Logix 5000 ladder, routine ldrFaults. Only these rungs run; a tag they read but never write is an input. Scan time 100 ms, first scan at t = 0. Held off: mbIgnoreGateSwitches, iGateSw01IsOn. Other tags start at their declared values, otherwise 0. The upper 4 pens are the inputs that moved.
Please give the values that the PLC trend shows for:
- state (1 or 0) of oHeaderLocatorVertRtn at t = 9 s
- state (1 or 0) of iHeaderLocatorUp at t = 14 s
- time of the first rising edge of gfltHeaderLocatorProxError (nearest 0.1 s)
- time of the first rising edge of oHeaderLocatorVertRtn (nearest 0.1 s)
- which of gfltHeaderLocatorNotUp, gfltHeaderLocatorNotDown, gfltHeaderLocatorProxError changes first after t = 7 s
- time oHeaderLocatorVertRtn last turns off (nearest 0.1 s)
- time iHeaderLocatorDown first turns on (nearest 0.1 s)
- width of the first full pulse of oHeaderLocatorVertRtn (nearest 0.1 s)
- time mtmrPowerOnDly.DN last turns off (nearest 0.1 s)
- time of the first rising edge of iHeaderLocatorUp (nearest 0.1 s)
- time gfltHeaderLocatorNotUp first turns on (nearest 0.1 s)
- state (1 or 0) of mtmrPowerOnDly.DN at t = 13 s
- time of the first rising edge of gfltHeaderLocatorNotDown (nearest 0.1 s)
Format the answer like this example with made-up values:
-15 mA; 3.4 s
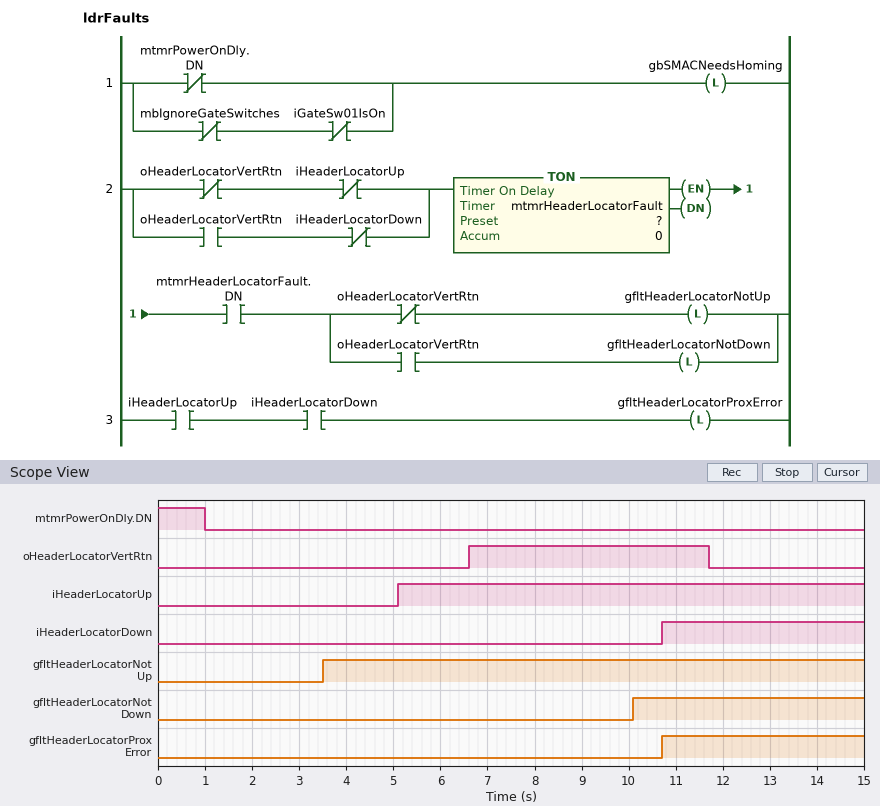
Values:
1; 1; 10.7 s; 6.6 s; gfltHeaderLocatorNotDown; 11.7 s; 10.7 s; 5.1 s; 1.0 s; 5.1 s; 3.5 s; 0; 10.1 s
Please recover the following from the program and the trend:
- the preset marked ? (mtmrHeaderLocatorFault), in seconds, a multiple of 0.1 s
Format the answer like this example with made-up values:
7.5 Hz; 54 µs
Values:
3.5 s
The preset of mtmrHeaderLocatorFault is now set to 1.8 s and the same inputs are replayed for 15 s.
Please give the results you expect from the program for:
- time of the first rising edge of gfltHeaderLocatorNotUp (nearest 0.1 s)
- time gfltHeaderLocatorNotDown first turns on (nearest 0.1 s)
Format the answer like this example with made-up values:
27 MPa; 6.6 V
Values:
1.8 s; 8.4 s
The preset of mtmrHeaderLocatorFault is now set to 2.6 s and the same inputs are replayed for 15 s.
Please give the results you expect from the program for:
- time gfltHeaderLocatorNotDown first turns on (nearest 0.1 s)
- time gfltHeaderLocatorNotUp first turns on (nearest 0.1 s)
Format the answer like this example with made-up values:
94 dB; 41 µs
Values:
9.2 s; 2.6 s
